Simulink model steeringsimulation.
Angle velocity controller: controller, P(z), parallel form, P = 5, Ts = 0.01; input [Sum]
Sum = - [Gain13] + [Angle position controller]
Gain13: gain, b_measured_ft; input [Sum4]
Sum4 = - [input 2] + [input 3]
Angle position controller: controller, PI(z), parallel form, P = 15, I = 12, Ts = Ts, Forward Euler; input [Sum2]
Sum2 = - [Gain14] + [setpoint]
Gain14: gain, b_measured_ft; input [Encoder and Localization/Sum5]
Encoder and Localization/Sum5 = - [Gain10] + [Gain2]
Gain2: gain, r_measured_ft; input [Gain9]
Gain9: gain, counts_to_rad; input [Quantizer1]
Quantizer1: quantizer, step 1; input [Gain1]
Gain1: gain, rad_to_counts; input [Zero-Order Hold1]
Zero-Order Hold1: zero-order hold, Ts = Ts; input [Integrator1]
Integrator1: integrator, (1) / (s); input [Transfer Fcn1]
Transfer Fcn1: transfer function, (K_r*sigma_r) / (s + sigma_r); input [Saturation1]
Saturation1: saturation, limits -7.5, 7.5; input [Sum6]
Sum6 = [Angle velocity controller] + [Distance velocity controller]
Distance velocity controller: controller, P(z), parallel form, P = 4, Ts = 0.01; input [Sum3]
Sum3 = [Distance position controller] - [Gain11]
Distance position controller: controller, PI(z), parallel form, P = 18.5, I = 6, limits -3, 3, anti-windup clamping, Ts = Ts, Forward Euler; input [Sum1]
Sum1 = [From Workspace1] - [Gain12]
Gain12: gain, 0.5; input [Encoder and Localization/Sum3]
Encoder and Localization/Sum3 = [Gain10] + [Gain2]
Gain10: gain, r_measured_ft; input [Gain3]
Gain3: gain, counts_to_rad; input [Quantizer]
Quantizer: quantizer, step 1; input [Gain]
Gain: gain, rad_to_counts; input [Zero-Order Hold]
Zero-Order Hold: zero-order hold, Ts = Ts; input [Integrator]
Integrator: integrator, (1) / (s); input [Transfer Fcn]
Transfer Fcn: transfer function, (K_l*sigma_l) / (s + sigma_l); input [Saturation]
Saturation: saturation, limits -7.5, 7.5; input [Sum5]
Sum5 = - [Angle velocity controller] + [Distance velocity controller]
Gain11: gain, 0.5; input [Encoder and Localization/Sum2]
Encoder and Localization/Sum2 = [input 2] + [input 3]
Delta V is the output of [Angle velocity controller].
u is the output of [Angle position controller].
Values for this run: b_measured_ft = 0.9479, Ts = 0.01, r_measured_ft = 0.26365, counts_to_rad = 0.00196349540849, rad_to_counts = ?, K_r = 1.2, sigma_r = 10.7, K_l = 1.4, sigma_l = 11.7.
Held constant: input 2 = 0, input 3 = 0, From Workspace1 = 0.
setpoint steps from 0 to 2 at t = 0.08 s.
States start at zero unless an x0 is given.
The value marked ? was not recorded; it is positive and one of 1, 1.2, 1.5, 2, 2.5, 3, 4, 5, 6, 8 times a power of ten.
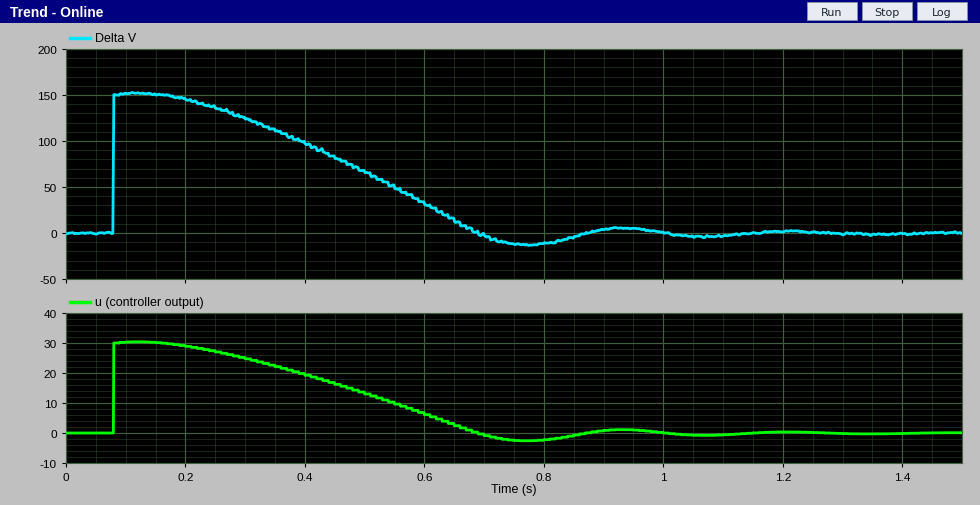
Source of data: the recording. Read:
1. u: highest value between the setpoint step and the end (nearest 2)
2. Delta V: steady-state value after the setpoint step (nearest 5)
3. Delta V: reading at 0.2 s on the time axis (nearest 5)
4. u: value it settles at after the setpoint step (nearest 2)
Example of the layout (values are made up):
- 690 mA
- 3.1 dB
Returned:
- 30
- 0
- 145
- 0
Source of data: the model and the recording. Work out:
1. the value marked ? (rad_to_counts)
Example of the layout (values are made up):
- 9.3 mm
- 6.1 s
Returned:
- 500
